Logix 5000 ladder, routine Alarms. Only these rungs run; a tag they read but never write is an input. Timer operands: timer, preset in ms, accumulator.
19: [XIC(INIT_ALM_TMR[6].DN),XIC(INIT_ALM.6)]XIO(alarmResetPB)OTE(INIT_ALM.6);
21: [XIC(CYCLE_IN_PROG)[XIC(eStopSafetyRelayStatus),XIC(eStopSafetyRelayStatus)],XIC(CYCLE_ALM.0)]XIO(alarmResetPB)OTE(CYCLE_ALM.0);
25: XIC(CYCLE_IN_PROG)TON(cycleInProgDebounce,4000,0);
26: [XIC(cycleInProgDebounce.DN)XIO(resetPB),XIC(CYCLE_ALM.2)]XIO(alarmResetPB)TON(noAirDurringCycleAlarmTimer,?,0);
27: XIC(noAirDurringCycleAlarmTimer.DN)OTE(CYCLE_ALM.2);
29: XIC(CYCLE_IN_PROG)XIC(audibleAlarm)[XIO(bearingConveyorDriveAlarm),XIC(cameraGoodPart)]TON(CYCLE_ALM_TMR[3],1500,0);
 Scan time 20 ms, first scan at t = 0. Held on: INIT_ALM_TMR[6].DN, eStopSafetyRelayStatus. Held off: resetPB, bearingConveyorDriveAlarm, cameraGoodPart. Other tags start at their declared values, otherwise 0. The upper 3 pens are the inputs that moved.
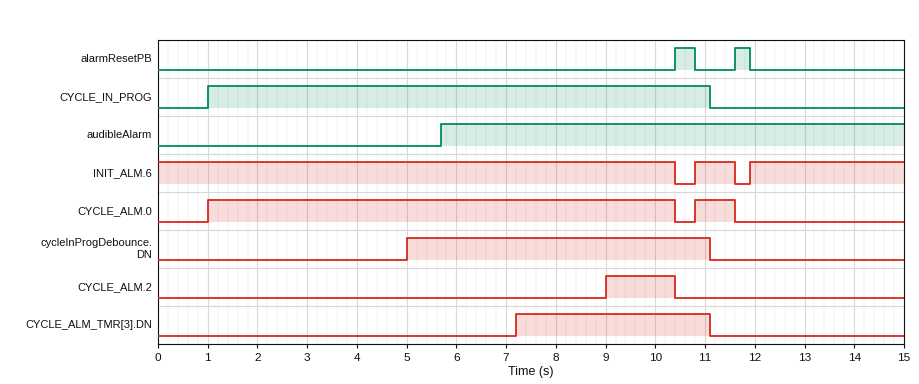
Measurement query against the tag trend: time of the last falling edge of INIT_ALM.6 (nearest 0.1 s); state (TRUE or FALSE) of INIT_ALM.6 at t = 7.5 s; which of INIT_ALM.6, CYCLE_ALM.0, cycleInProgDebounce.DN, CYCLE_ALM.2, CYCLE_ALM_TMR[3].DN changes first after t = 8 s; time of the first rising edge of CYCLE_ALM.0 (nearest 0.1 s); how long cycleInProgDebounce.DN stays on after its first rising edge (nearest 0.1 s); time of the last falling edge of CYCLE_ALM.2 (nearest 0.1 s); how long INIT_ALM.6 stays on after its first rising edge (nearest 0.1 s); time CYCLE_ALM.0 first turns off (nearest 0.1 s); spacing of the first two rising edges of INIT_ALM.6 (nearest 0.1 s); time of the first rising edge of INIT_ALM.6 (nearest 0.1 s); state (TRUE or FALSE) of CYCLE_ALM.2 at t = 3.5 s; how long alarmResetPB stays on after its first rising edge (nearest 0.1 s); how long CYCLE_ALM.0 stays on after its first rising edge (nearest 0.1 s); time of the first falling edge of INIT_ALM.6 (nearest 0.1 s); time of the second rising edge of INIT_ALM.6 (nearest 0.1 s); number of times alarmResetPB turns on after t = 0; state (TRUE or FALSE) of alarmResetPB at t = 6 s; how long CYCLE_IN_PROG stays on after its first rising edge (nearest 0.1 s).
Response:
11.6 s
TRUE
CYCLE_ALM.2
1.0 s
6.1 s
10.4 s
0.8 s
10.4 s
1.1 s
10.8 s
FALSE
0.4 s
9.4 s
10.4 s
11.9 s
2
FALSE
10.1 s
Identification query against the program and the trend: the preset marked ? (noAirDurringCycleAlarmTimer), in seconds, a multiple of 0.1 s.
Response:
4.0 s
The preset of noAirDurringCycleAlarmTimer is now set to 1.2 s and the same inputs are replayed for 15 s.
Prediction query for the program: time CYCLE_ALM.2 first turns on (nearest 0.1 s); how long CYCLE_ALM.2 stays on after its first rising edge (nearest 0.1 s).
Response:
6.2 s
4.2 s
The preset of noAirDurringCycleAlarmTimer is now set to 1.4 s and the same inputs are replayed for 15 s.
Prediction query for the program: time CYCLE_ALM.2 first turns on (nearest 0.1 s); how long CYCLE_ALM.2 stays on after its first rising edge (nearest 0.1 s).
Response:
6.4 s
4.0 s
